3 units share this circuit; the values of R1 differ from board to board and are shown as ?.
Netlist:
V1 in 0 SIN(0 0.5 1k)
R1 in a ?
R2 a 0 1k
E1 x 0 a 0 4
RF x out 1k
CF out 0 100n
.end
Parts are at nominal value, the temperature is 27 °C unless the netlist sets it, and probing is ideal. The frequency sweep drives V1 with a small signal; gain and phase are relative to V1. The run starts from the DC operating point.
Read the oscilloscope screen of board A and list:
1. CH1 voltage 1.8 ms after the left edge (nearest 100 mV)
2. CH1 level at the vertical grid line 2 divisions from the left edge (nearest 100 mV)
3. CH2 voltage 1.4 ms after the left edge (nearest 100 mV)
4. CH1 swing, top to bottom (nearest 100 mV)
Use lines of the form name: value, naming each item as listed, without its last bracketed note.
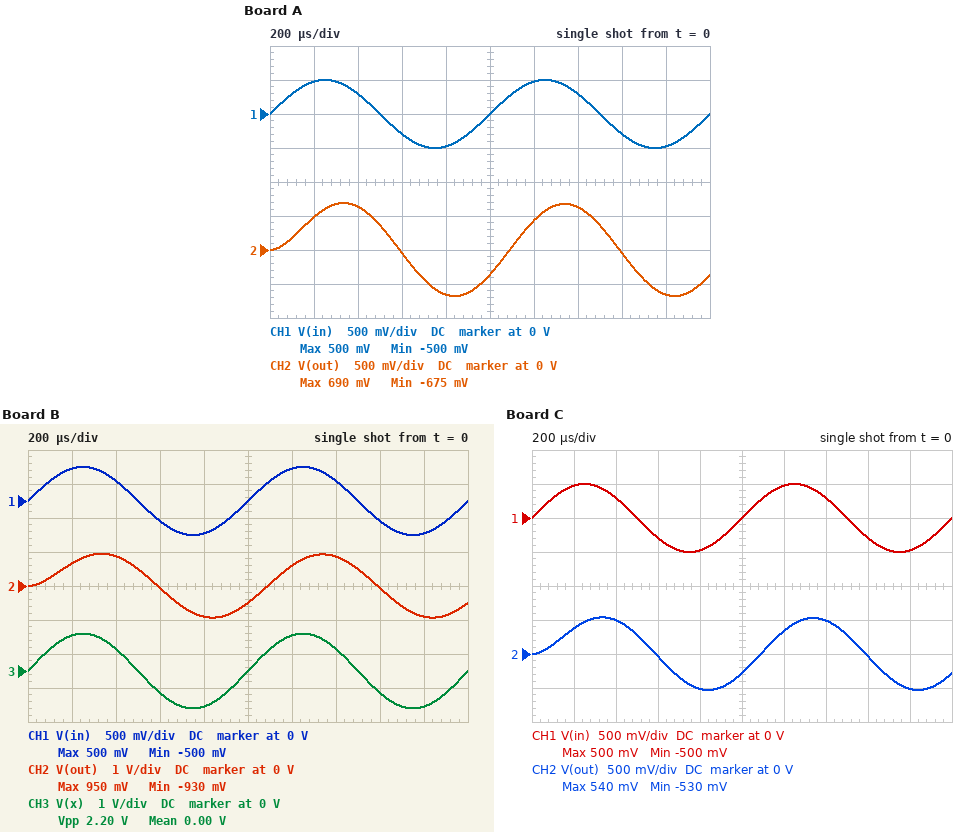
CH1 voltage 1.8 ms after the left edge: -500 mV
CH1 level at the vertical grid line 2 divisions from the left edge: 300 mV
CH2 voltage 1.4 ms after the left edge: 600 mV
CH1 swing, top to bottom: 1.0 V
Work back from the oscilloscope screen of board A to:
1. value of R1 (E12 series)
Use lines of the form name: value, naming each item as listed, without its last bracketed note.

value of R1: 1.5 kΩ
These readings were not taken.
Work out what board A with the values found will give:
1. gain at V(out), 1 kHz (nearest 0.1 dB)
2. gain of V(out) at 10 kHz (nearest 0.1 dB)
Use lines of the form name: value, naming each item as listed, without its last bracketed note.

gain at V(out), 1 kHz: 2.6 dB
gain of V(out) at 10 kHz: -12.0 dB
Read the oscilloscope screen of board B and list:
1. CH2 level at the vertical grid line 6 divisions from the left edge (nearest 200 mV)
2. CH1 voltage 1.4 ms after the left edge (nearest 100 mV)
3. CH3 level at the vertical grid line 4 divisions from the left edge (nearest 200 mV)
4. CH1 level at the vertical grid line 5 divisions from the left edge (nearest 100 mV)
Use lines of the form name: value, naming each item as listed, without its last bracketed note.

CH2 level at the vertical grid line 6 divisions from the left edge: 600 mV
CH1 voltage 1.4 ms after the left edge: 300 mV
CH3 level at the vertical grid line 4 divisions from the left edge: -1.0 V
CH1 level at the vertical grid line 5 divisions from the left edge: 0 V
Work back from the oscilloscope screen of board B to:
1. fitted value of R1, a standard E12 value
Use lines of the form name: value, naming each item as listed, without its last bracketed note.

fitted value of R1, a standard E12 value: 820 Ω
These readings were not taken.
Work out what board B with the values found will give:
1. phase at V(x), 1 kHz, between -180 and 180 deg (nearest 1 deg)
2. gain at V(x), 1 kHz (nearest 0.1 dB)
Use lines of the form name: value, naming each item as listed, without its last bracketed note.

phase at V(x), 1 kHz, between -180 and 180 deg: 0 deg
gain at V(x), 1 kHz: 6.8 dB
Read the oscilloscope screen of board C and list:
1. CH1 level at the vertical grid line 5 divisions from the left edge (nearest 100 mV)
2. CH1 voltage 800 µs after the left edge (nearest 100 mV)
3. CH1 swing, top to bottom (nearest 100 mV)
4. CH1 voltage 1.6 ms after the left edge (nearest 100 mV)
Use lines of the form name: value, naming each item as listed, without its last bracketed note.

CH1 level at the vertical grid line 5 divisions from the left edge: 0 V
CH1 voltage 800 µs after the left edge: -500 mV
CH1 swing, top to bottom: 1.0 V
CH1 voltage 1.6 ms after the left edge: -300 mV
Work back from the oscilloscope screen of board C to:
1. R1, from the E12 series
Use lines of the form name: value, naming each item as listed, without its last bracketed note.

R1, from the E12 series: 2.2 kΩ
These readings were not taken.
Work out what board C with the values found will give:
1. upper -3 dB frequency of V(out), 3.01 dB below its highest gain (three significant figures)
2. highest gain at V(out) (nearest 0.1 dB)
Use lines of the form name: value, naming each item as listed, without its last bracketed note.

upper -3 dB frequency of V(out), 3.01 dB below its highest gain: 1.59 kHz
highest gain at V(out): 1.9 dB
